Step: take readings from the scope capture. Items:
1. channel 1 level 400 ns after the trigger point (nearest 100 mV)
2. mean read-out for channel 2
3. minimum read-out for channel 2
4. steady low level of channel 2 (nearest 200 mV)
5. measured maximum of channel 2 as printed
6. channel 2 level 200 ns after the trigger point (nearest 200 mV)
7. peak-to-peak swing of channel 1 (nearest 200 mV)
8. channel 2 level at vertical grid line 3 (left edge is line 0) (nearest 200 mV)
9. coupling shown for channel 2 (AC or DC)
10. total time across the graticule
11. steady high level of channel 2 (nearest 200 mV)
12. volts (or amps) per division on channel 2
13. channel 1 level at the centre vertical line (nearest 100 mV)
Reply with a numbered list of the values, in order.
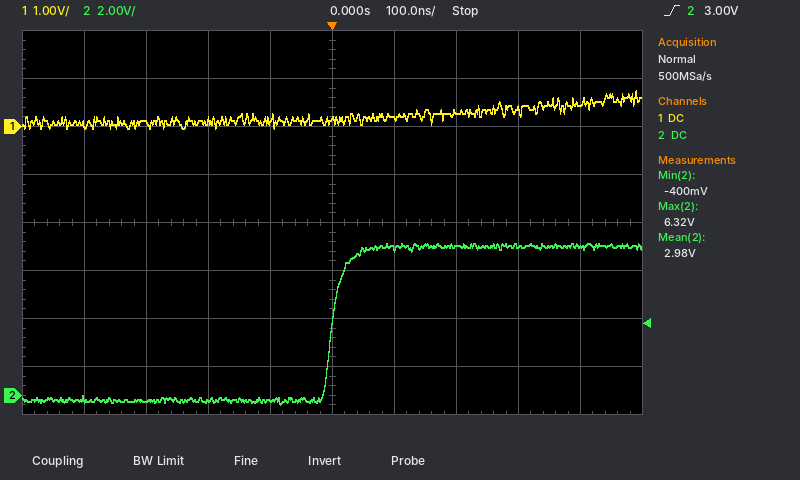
1. 500 mV
2. 2.98 V
3. -400 mV
4. -200 mV
5. 6.32 V
6. 6.2 V
7. 800 mV
8. -200 mV
9. DC
10. 1 µs
11. 6.2 V
12. 2 V
13. 100 mV
